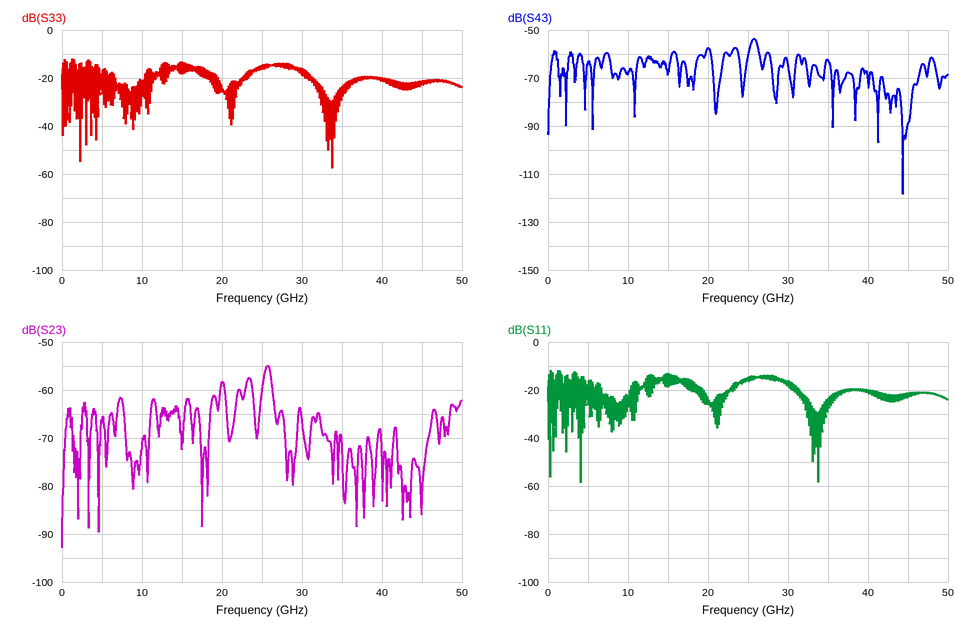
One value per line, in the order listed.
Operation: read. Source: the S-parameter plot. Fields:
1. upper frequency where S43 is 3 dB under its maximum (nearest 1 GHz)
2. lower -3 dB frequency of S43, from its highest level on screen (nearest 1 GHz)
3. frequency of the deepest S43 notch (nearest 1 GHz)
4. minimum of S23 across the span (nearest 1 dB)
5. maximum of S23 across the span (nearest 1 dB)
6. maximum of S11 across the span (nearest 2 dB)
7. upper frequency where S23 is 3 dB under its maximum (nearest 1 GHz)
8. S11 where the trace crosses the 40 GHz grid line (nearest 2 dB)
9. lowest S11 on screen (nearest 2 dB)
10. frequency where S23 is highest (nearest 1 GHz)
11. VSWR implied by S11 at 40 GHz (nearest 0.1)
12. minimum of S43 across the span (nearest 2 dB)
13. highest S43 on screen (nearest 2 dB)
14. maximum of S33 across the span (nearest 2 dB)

26 GHz
25 GHz
44 GHz
-93 dB
-55 dB
-12 dB
26 GHz
-20 dB
-58 dB
26 GHz
1.2
-118 dB
-54 dB
-12 dB
